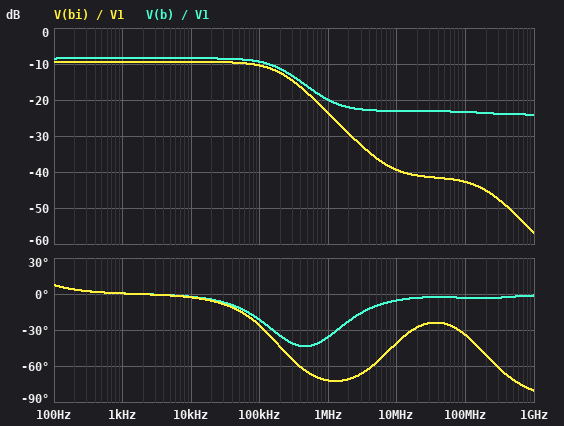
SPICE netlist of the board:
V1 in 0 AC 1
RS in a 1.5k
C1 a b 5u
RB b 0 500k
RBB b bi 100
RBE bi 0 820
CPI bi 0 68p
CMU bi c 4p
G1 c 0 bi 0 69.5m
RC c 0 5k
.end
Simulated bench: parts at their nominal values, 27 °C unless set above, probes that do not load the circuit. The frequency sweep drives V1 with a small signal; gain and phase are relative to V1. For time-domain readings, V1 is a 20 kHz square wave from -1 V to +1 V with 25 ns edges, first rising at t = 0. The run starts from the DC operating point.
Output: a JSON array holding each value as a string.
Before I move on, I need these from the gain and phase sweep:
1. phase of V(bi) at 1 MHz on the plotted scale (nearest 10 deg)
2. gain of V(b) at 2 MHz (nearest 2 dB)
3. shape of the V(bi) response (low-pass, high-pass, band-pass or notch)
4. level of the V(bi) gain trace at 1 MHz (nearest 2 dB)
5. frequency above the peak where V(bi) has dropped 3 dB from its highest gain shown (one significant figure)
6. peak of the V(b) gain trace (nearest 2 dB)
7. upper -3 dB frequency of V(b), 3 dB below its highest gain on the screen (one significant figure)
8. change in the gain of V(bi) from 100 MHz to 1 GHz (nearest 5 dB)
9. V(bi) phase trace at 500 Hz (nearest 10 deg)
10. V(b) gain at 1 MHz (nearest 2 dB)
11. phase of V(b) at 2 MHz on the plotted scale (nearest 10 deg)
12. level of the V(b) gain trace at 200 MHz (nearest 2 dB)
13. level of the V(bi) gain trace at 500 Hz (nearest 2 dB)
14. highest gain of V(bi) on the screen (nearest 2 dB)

["-70 deg", "-22 dB", "low-pass", "-24 dB", "200 kHz", "-8 dB", "200 kHz", "-15 dB", "0 deg", "-20 dB", "-20 deg", "-24 dB", "-10 dB", "-10 dB"]
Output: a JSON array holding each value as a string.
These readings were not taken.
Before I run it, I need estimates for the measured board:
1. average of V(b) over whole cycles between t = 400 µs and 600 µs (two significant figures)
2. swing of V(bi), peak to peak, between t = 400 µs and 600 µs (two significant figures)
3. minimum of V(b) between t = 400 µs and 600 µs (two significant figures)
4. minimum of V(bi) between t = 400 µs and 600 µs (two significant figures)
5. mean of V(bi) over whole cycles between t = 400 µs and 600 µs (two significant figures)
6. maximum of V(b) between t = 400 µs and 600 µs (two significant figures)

["360 mV", "680 mV", "-18 mV", "-16 mV", "320 mV", "750 mV"]
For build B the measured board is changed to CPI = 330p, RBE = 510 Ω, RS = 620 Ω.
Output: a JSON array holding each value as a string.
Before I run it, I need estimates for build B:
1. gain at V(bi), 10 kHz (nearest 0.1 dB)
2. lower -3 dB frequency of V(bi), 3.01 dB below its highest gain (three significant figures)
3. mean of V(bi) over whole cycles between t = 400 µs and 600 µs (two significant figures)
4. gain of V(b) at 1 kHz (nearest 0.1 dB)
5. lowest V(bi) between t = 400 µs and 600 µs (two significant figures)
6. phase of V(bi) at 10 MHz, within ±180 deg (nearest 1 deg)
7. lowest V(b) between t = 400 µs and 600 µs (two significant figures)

["-7.7 dB", "25.9 Hz", "380 mV", "-6.1 dB", "-39 mV", "-50 deg", "-46 mV"]
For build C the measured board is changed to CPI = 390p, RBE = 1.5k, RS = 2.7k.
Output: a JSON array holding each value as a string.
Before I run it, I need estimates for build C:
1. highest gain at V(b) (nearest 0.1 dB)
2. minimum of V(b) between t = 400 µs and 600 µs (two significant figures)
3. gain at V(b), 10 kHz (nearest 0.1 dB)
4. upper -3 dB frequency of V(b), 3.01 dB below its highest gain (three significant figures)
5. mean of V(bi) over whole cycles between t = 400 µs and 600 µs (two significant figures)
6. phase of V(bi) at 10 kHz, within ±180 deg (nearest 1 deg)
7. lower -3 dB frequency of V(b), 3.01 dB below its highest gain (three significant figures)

["-8.6 dB", "-10 mV", "-8.7 dB", "91.7 kHz", "340 mV", "-6 deg", "7.41 Hz"]
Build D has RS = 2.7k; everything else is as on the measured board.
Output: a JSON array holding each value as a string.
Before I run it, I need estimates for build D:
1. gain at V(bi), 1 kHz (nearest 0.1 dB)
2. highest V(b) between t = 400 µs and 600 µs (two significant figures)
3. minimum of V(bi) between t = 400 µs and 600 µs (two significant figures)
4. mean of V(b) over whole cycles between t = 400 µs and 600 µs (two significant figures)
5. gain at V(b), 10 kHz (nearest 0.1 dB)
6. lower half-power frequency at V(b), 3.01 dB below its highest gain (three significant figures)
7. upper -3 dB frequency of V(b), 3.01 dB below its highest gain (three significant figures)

["-12.9 dB", "500 mV", "-7.4 mV", "250 mV", "-11.9 dB", "8.80 Hz", "173 kHz"]
